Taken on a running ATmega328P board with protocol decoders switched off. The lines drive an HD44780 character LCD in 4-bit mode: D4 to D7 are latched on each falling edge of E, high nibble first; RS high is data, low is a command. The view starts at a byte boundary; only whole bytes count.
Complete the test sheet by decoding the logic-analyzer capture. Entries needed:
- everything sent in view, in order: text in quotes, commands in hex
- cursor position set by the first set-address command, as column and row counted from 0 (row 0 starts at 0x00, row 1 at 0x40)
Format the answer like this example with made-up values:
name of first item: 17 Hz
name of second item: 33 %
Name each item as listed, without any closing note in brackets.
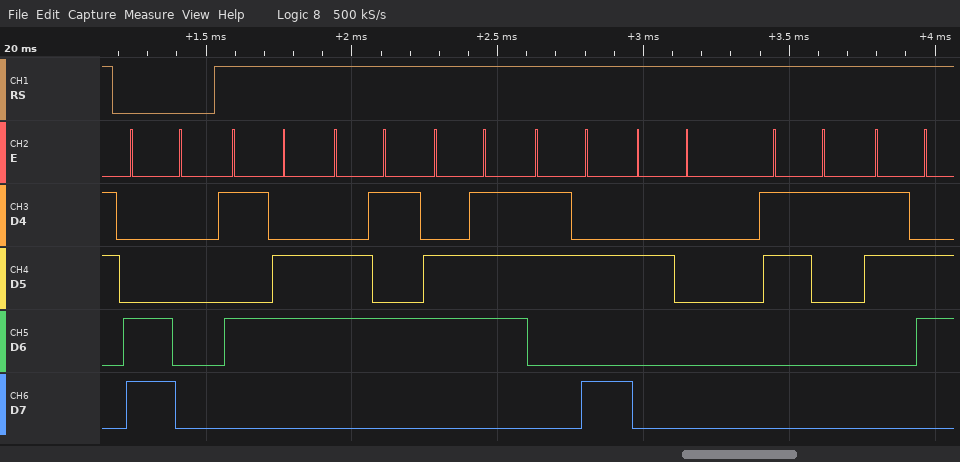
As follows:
everything sent in view, in order: text in quotes, commands in hex: 0xC0 "Veg: 16"
cursor position set by the first set-address command, as column and row counted from 0: column 0, row 1
